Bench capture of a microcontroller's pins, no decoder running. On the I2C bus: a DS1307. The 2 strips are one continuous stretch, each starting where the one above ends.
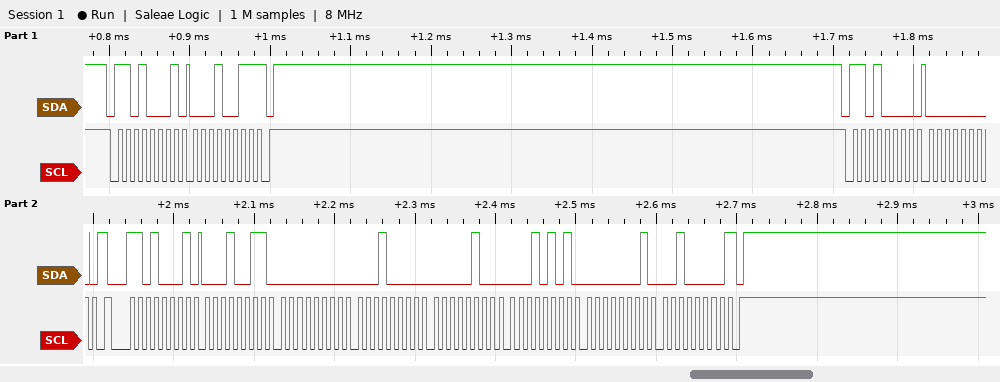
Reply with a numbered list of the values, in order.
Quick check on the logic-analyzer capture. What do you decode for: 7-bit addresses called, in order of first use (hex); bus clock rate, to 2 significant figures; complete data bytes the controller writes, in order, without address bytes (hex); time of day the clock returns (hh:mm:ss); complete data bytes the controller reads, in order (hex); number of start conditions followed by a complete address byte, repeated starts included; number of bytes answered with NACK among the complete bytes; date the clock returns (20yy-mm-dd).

1. 0x68
2. 100 kHz
3. 00
4. 10:00:13
5. 13 13 00 10 04 15 01 20
6. 3
7. 2
8. 2020-01-15
